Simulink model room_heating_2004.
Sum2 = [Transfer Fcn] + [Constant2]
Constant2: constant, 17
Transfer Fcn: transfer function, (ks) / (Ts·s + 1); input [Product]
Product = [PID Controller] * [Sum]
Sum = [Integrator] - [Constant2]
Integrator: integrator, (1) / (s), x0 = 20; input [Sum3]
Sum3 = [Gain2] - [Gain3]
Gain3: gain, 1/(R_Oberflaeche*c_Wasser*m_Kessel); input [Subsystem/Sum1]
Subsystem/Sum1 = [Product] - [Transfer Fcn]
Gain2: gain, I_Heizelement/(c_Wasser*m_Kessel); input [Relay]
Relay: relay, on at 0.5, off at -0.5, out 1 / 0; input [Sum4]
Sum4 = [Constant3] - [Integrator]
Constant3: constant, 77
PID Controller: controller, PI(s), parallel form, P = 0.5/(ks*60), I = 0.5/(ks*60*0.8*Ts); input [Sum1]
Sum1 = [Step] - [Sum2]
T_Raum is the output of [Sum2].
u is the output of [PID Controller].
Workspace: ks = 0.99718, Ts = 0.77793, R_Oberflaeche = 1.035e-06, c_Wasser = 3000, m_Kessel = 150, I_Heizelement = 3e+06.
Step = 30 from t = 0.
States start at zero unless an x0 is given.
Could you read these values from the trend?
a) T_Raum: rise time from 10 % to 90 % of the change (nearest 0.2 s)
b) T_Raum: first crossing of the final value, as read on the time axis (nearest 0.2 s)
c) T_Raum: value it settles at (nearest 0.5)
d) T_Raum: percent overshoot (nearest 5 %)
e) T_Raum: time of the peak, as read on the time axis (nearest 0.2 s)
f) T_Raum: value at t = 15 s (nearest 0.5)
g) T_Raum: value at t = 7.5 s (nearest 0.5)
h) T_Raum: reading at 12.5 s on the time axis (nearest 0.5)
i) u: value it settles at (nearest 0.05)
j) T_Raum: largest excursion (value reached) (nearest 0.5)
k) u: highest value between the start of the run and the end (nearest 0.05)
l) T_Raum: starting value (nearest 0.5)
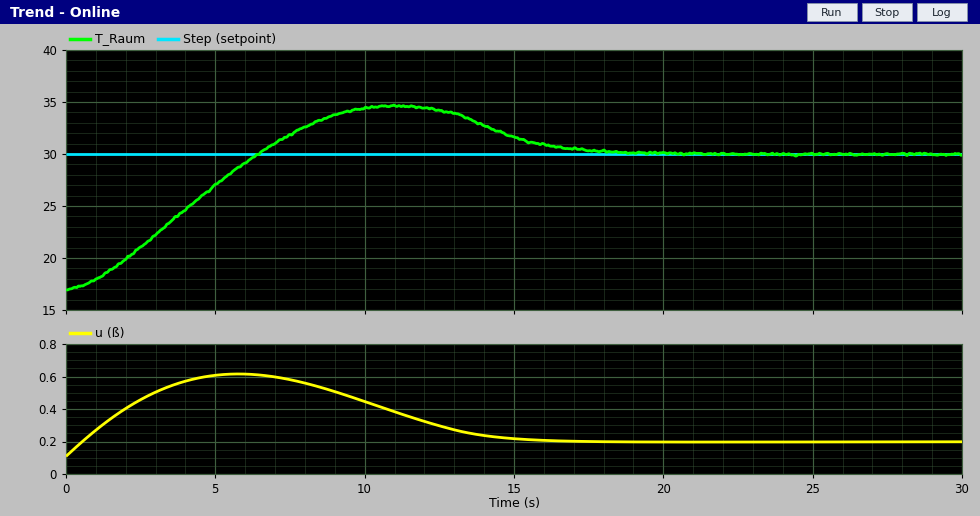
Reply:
4.6 s
6.4 s
30.0
35 %
11.0 s
31.5
32.0
34.0
0.20
34.5
0.60
17.0
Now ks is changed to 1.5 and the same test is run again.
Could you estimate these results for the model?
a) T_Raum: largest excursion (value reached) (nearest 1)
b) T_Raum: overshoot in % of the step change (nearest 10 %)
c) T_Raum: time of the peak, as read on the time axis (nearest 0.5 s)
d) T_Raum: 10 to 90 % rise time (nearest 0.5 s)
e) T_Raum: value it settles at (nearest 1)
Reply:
37
50 %
7.0 s
3.0 s
30
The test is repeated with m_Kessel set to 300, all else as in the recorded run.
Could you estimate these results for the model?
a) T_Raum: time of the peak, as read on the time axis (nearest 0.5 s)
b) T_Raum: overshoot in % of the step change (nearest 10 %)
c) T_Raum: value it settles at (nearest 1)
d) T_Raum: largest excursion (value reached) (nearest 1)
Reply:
13.5 s
30 %
30
34
